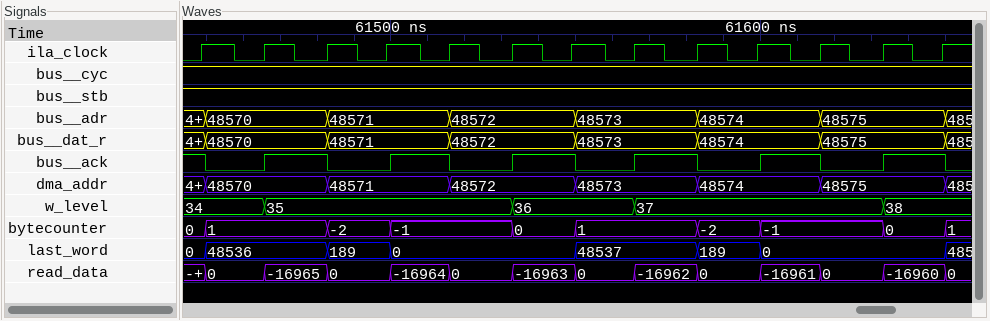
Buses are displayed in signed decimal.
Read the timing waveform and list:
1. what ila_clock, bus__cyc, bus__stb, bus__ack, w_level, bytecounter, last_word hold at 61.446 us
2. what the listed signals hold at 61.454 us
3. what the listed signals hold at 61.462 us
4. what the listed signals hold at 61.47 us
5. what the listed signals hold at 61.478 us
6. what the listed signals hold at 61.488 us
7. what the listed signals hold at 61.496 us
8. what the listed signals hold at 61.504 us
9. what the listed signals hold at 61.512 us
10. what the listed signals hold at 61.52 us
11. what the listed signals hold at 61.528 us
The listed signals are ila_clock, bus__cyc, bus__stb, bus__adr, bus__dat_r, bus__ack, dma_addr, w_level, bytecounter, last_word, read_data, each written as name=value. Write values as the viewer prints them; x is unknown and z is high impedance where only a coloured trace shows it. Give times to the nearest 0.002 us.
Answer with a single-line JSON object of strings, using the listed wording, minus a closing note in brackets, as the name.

{"what ila_clock, bus__cyc, bus__stb, bus__ack, w_level, bytecounter, last_word hold at 61.446 us": "ila_clock=0, bus__cyc=1, bus__stb=1, bus__ack=1, w_level=34, bytecounter=0, last_word=0", "what the listed signals hold at 61.454 us": "ila_clock=1, bus__cyc=1, bus__stb=1, bus__adr=48570, bus__dat_r=48570, bus__ack=0, dma_addr=48570, w_level=34, bytecounter=1, last_word=48536, read_data=0", "what the listed signals hold at 61.462 us": "ila_clock=0, bus__cyc=1, bus__stb=1, bus__adr=48570, bus__dat_r=48570, bus__ack=0, dma_addr=48570, w_level=34, bytecounter=1, last_word=48536, read_data=0", "what the listed signals hold at 61.47 us": "ila_clock=1, bus__cyc=1, bus__stb=1, bus__adr=48570, bus__dat_r=48570, bus__ack=1, dma_addr=48570, w_level=35, bytecounter=1, last_word=48536, read_data=-16965", "what the listed signals hold at 61.478 us": "ila_clock=0, bus__cyc=1, bus__stb=1, bus__adr=48570, bus__dat_r=48570, bus__ack=1, dma_addr=48570, w_level=35, bytecounter=1, last_word=48536, read_data=-16965", "what the listed signals hold at 61.488 us": "ila_clock=1, bus__cyc=1, bus__stb=1, bus__adr=48571, bus__dat_r=48571, bus__ack=0, dma_addr=48571, w_level=35, bytecounter=-2, last_word=189, read_data=0", "what the listed signals hold at 61.496 us": "ila_clock=0, bus__cyc=1, bus__stb=1, bus__adr=48571, bus__dat_r=48571, bus__ack=0, dma_addr=48571, w_level=35, bytecounter=-2, last_word=189, read_data=0", "what the listed signals hold at 61.504 us": "ila_clock=1, bus__cyc=1, bus__stb=1, bus__adr=48571, bus__dat_r=48571, bus__ack=1, dma_addr=48571, w_level=35, bytecounter=-1, last_word=0, read_data=-16964", "what the listed signals hold at 61.512 us": "ila_clock=0, bus__cyc=1, bus__stb=1, bus__adr=48571, bus__dat_r=48571, bus__ack=1, dma_addr=48571, w_level=35, bytecounter=-1, last_word=0, read_data=-16964", "what the listed signals hold at 61.52 us": "ila_clock=1, bus__cyc=1, bus__stb=1, bus__adr=48572, bus__dat_r=48572, bus__ack=0, dma_addr=48572, w_level=35, bytecounter=-1, last_word=0, read_data=0", "what the listed signals hold at 61.528 us": "ila_clock=0, bus__cyc=1, bus__stb=1, bus__adr=48572, bus__dat_r=48572, bus__ack=0, dma_addr=48572, w_level=35, bytecounter=-1, last_word=0, read_data=0"}
